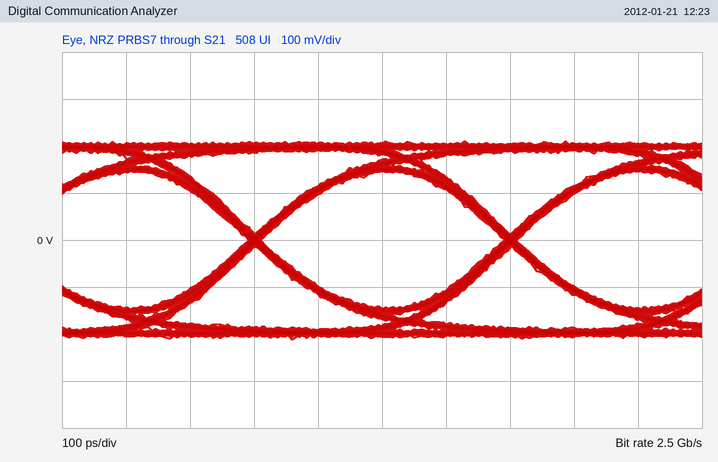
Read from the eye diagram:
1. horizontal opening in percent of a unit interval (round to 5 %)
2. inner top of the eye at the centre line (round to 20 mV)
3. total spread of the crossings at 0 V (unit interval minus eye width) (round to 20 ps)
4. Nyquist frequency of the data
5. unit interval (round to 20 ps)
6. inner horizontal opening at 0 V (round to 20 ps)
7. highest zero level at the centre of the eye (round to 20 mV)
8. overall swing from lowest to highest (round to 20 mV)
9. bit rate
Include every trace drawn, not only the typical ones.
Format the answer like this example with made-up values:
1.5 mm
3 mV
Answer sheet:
95 %
140 mV
20 ps
1.25 GHz
400 ps
380 ps
-140 mV
420 mV
2.5 Gb/s
